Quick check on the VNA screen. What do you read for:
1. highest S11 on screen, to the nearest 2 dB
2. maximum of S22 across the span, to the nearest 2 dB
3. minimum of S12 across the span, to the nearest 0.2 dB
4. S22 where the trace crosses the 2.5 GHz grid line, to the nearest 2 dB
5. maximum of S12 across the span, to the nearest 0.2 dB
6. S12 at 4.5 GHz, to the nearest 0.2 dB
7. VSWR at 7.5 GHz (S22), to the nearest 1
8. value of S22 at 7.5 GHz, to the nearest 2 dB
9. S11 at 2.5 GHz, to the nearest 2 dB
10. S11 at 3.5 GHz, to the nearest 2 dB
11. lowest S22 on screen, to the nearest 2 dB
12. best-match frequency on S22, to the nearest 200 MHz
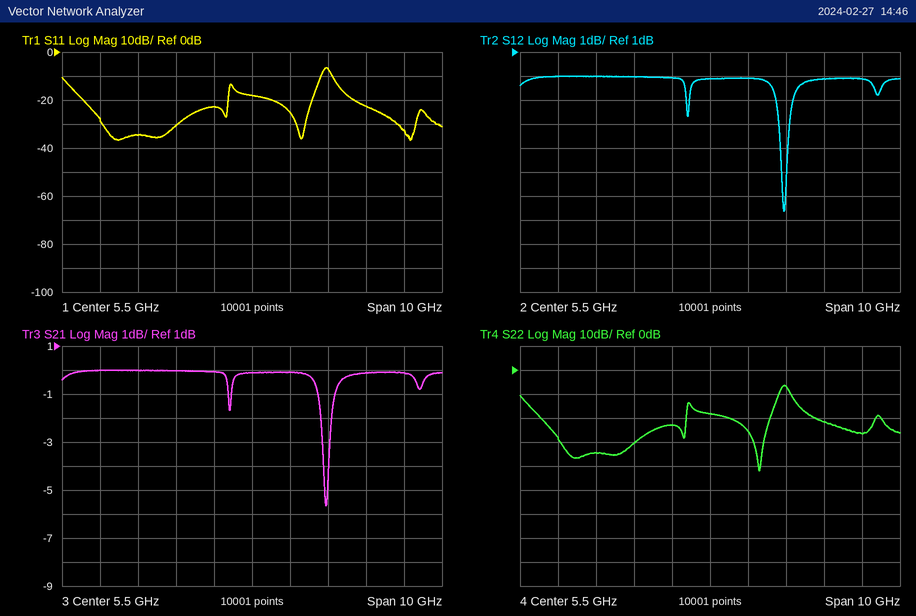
-6 dB
-6 dB
-5.6 dB
-34 dB
0.0 dB
0.0 dB
3
-6 dB
-34 dB
-30 dB
-42 dB
6.8 GHz
